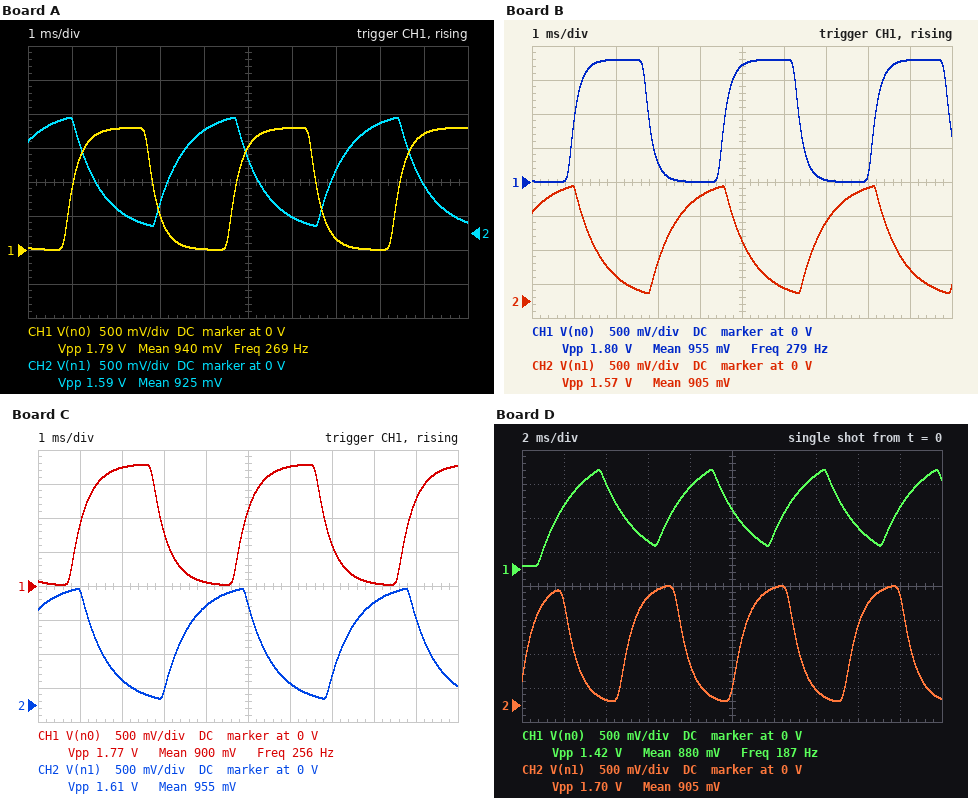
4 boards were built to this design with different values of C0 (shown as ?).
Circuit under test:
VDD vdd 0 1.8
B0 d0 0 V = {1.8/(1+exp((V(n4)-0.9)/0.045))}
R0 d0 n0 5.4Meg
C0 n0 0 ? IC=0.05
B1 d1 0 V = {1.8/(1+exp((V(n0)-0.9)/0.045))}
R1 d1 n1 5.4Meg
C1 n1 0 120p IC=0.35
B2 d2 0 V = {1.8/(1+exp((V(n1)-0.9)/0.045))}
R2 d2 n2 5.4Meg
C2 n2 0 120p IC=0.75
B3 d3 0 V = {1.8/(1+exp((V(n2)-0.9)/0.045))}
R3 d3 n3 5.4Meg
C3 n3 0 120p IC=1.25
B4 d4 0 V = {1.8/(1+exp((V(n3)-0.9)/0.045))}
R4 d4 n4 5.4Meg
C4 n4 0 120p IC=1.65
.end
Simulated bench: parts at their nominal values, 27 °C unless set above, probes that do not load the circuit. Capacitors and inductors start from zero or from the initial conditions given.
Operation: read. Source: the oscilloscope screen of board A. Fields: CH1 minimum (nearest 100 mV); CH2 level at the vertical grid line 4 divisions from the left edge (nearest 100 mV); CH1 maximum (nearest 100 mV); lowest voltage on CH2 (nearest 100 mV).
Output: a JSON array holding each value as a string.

["0 V", "1.5 V", "1.8 V", "100 mV"]
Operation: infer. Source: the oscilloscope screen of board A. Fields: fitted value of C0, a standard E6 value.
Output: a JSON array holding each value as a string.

["47 pF"]
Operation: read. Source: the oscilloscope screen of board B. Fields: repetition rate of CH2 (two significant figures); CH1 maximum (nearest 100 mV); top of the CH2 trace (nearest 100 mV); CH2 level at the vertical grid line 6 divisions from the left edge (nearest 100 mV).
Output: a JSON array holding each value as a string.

["280 Hz", "1.8 V", "1.7 V", "200 mV"]
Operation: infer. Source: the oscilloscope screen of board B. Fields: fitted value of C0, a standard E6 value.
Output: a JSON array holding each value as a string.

["33 pF"]
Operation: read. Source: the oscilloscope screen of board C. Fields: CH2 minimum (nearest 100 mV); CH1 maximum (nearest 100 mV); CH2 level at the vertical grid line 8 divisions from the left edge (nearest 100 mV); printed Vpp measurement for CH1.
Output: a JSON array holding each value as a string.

["100 mV", "1.8 V", "1.5 V", "1.77 V"]
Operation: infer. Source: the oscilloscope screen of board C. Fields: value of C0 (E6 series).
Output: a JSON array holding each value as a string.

["68 pF"]
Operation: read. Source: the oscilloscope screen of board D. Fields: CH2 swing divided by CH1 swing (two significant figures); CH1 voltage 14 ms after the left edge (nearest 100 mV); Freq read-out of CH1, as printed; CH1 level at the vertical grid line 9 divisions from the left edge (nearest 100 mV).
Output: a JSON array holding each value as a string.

["1.2", "1.4 V", "187 Hz", "900 mV"]
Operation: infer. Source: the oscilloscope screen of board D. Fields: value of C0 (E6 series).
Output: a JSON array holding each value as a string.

["330 pF"]
